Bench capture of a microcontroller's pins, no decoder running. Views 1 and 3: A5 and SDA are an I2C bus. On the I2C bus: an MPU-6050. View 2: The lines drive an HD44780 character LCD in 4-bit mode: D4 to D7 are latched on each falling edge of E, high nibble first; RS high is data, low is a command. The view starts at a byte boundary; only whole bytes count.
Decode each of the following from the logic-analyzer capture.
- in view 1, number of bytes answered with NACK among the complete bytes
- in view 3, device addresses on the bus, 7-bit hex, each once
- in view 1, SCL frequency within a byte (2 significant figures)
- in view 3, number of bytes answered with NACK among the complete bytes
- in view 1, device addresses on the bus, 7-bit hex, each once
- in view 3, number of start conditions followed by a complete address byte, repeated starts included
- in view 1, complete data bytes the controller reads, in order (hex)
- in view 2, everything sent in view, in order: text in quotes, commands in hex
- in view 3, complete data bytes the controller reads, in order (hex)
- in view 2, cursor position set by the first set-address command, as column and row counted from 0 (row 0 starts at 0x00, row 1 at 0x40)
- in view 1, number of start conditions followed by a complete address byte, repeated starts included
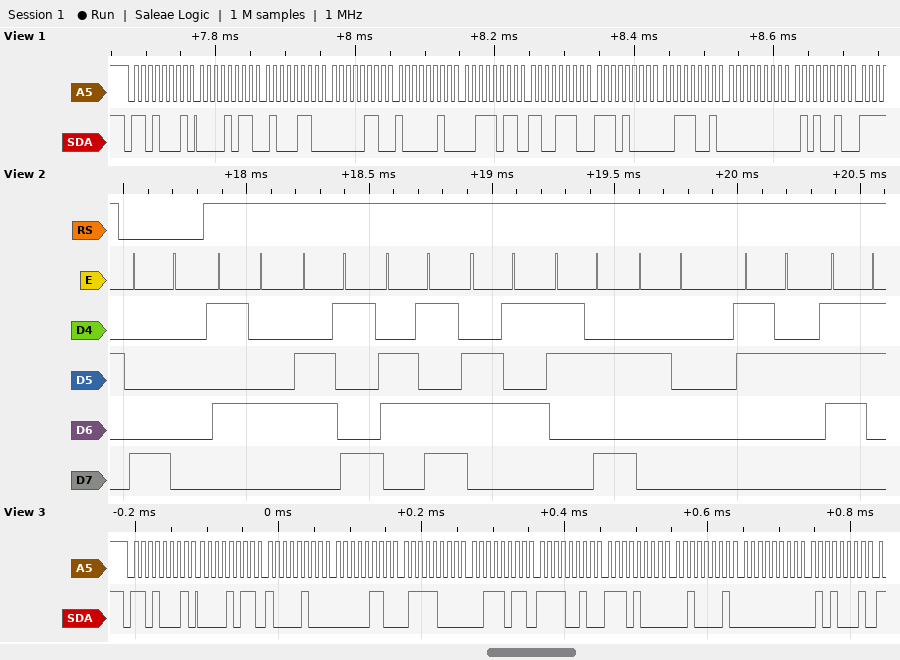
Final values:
0
0x68
100 kHz
0
0x68
1
0B 46 06 82 3B CE E8 39 00 52
0x80 "Time: 2s"
0B 84 06 78 3B F2 E8 21 00 51
column 0, row 0
1
